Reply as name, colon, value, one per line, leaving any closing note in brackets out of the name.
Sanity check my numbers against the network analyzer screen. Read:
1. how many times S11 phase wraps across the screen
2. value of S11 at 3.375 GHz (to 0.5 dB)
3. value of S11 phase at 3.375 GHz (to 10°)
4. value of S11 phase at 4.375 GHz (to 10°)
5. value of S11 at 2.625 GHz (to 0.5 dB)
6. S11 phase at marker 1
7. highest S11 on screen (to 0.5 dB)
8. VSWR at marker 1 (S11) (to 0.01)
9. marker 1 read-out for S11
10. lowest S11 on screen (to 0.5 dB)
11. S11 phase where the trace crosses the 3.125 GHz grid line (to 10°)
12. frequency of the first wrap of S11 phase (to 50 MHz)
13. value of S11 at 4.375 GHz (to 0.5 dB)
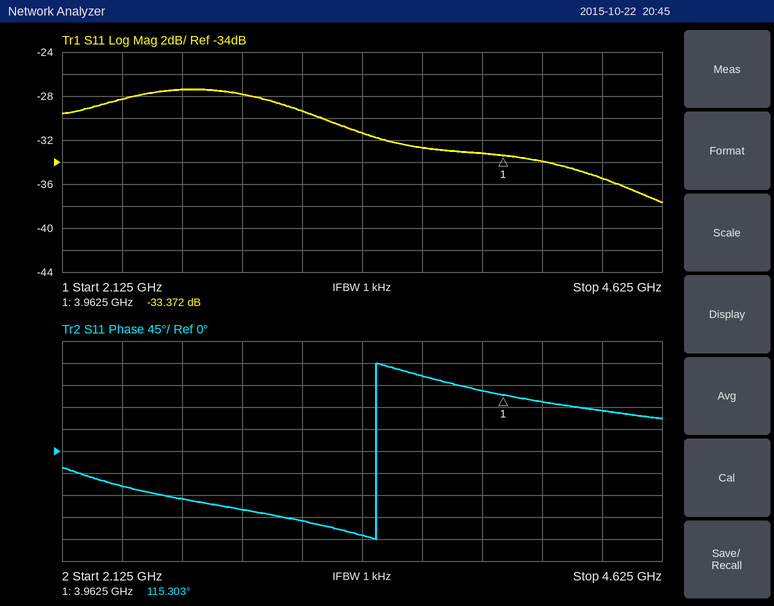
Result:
how many times S11 phase wraps across the screen: 1
value of S11 at 3.375 GHz: -31.5 dB
value of S11 phase at 3.375 GHz: -170°
value of S11 phase at 4.375 GHz: 80°
value of S11 at 2.625 GHz: -27.5 dB
S11 phase at marker 1: 115.303°
highest S11 on screen: -27.5 dB
VSWR at marker 1 (S11): 1.04
marker 1 read-out for S11: -33.372 dB
lowest S11 on screen: -37.5 dB
S11 phase where the trace crosses the 3.125 GHz grid line: -140°
frequency of the first wrap of S11 phase: 3.45 GHz
value of S11 at 4.375 GHz: -35.5 dB
